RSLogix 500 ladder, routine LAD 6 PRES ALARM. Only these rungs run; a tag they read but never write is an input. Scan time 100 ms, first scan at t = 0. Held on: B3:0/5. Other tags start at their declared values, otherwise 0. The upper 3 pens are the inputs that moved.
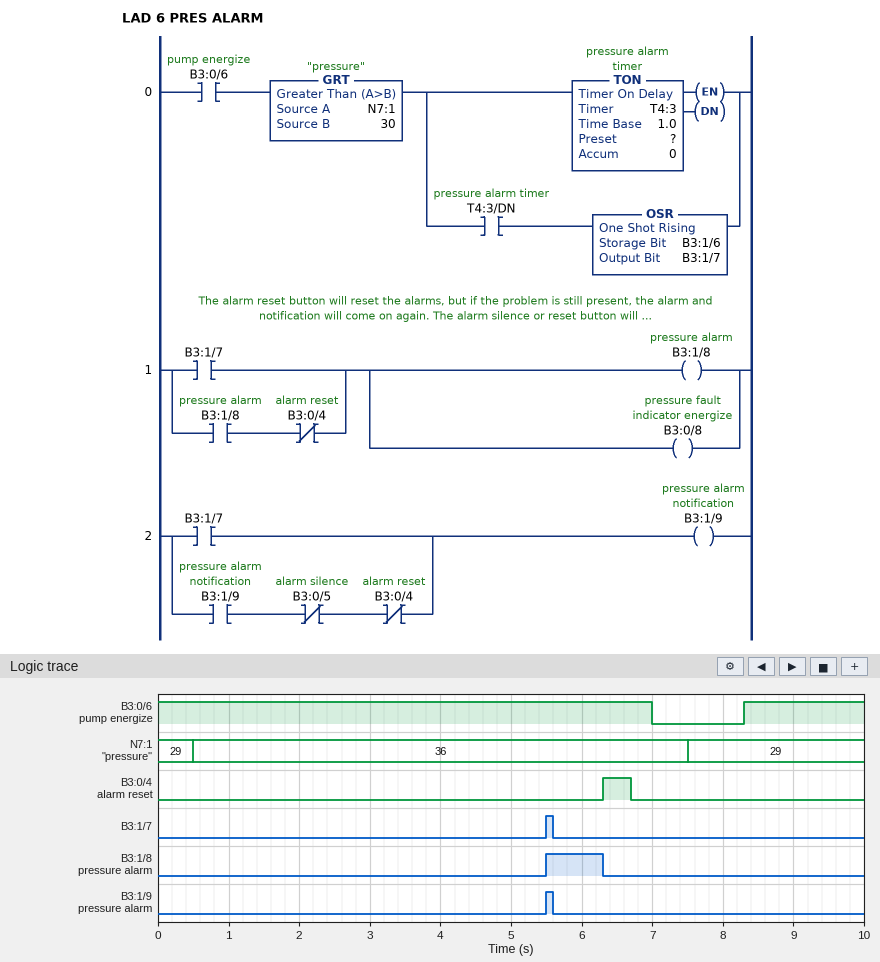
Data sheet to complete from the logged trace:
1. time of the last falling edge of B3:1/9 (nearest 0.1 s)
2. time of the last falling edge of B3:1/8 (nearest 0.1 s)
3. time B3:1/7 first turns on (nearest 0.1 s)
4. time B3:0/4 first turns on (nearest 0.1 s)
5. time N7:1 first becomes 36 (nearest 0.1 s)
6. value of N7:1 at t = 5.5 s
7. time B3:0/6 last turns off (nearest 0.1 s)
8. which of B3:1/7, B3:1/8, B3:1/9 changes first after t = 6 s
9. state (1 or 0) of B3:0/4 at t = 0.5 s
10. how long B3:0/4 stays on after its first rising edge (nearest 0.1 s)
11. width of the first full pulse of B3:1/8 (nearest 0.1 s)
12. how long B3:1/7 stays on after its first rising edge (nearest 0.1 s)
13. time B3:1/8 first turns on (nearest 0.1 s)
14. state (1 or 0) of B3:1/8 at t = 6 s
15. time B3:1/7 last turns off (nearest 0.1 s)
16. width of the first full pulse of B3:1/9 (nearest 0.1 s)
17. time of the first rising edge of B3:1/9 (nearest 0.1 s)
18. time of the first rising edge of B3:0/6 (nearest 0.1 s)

5.6 s
6.3 s
5.5 s
6.3 s
0.5 s
36
7.0 s
B3:1/8
0
0.4 s
0.8 s
0.1 s
5.5 s
1
5.6 s
0.1 s
5.5 s
8.3 s
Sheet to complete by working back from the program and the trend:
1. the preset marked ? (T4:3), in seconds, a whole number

5 s
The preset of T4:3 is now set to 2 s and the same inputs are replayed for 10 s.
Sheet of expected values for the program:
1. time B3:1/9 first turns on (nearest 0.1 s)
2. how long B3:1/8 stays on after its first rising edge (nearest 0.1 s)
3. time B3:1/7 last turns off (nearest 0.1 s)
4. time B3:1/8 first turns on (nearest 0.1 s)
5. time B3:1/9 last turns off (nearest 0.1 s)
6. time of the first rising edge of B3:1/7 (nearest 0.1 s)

2.5 s
3.8 s
2.6 s
2.5 s
2.6 s
2.5 s
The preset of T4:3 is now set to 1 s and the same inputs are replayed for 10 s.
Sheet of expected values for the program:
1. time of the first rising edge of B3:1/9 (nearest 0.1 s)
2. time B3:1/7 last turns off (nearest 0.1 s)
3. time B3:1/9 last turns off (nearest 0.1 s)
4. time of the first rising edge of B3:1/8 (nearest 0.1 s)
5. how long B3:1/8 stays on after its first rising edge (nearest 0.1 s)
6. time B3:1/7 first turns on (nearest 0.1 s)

1.5 s
1.6 s
1.6 s
1.5 s
4.8 s
1.5 s
